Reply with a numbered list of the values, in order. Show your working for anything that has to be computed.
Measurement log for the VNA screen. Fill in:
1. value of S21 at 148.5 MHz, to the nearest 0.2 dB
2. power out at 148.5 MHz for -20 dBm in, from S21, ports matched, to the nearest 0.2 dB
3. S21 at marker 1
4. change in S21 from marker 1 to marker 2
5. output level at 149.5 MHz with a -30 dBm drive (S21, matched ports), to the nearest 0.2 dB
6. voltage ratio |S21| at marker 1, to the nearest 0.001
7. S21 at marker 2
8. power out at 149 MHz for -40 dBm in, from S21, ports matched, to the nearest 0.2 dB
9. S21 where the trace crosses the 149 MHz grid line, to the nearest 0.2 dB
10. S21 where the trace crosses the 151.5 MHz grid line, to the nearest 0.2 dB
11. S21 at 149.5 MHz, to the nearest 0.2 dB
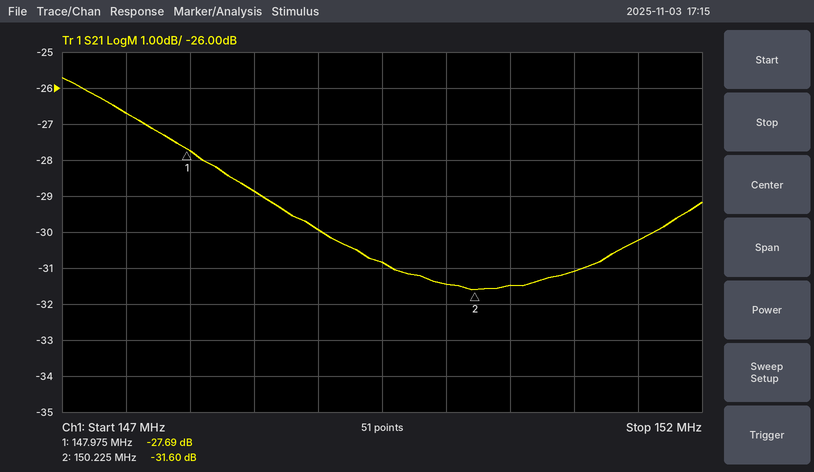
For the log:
1. -28.8 dB
2. -20 dBm + (-28.8 dB) = -48.8 dBm
3. -27.69 dB
4. -31.6 − (-27.69) = -3.91 dB
5. -30 dBm + (-30.8 dB) = -60.8 dBm
6. 10^(-27.69/20) ≈ 0.041
7. -31.60 dB
8. -40 dBm + (-30.0 dB) = -70.0 dBm
9. -30.0 dB
10. -30.2 dB
11. -30.8 dB
